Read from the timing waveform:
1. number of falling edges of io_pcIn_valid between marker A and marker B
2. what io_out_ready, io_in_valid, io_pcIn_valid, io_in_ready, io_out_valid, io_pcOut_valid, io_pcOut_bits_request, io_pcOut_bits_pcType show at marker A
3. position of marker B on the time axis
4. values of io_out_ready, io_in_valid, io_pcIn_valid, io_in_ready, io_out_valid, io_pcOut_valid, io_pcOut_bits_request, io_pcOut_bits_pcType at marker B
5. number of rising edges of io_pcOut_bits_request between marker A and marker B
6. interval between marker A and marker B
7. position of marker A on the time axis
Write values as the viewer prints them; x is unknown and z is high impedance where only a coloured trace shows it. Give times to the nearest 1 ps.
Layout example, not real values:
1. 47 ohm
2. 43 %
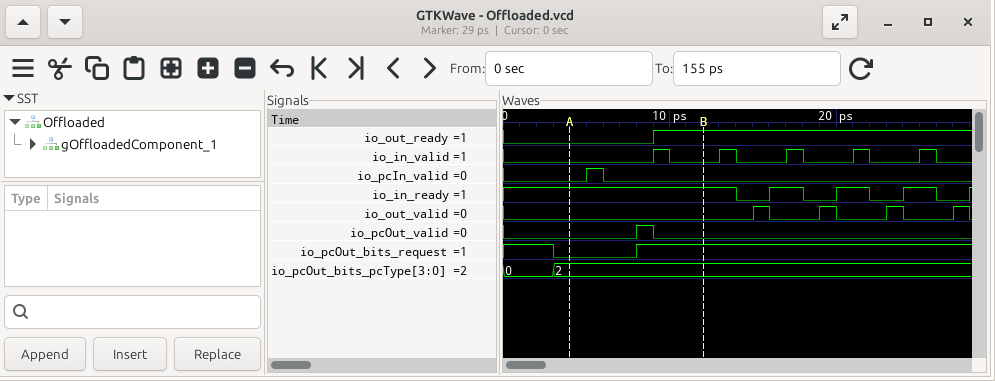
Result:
1. 1
2. io_out_ready=0, io_in_valid=0, io_pcIn_valid=0, io_in_ready=1, io_out_valid=0, io_pcOut_valid=0, io_pcOut_bits_request=0, io_pcOut_bits_pcType=2
3. 12 ps
4. io_out_ready=1, io_in_valid=0, io_pcIn_valid=0, io_in_ready=1, io_out_valid=0, io_pcOut_valid=0, io_pcOut_bits_request=1, io_pcOut_bits_pcType=2
5. 1
6. 8 ps
7. 4 ps
